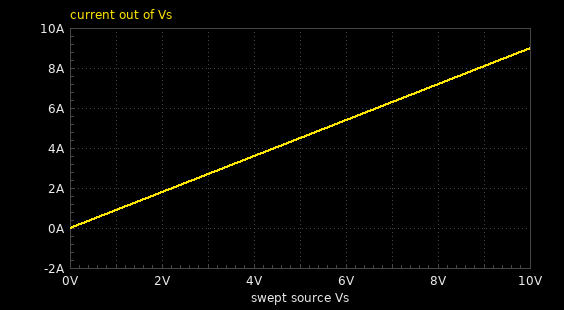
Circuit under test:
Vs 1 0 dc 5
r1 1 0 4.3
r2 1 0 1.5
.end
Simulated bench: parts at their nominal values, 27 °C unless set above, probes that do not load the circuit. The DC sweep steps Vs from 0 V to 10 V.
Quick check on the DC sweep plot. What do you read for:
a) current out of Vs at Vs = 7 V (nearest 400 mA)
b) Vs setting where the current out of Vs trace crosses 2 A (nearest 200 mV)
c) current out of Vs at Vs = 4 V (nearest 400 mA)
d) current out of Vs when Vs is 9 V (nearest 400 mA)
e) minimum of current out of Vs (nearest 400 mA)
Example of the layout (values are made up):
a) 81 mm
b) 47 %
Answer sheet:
a) 6.4 A
b) 2.2 V
c) 3.6 A
d) 8.0 A
e) 0 A
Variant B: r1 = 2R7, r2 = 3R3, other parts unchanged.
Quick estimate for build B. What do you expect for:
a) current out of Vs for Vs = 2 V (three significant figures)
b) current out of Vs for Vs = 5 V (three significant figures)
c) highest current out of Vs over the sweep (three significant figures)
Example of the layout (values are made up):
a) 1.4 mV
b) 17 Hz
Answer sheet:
a) 1.35 A
b) 3.37 A
c) 6.73 A
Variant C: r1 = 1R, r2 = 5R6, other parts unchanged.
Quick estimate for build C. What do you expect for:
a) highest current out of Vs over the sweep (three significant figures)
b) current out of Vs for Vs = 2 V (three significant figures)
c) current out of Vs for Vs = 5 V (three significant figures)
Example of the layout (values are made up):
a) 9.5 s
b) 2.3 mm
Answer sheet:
a) 11.8 A
b) 2.36 A
c) 5.89 A
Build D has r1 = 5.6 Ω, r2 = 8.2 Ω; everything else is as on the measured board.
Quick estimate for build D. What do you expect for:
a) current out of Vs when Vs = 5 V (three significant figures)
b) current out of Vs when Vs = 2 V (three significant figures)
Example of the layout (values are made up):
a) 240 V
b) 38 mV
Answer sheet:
a) 1.50 A
b) 601 mA
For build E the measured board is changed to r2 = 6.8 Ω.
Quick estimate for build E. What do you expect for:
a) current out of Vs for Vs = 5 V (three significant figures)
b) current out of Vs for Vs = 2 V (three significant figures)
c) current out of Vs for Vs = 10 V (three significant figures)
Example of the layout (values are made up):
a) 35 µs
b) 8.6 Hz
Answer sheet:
a) 1.90 A
b) 759 mA
c) 3.80 A
